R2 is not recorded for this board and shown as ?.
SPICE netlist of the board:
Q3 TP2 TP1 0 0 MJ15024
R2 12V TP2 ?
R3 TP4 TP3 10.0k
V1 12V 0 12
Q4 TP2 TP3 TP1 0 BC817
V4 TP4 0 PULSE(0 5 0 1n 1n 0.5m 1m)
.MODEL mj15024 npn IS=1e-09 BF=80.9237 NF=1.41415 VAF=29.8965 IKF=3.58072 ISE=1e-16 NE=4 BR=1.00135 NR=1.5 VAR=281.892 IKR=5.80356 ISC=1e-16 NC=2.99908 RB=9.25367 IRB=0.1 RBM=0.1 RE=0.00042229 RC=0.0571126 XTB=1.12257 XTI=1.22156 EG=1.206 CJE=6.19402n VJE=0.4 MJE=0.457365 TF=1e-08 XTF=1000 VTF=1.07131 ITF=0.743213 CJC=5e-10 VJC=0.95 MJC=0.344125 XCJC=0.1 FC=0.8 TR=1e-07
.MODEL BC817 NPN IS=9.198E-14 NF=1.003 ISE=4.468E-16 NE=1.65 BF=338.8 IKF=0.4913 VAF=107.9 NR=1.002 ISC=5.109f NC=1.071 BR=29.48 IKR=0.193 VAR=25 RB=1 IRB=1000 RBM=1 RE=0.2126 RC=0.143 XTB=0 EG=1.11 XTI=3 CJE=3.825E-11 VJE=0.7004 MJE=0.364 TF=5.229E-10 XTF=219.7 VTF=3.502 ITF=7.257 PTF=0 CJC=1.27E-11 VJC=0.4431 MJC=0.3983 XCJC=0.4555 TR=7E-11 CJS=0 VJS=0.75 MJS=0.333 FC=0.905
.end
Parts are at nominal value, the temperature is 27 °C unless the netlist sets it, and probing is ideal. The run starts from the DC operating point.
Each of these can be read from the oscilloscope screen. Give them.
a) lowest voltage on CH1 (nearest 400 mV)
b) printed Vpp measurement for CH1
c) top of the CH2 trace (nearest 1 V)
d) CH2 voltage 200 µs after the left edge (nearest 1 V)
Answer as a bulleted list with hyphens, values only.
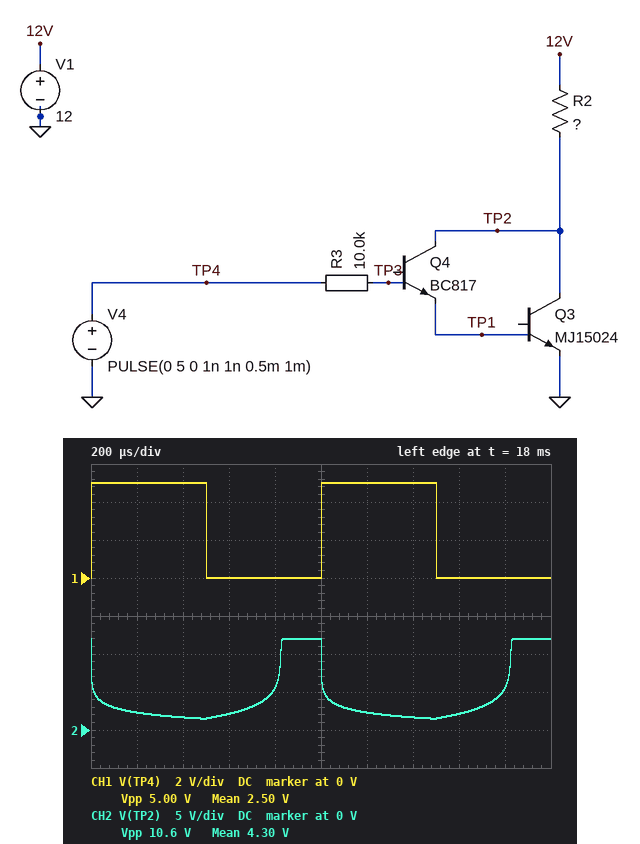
- 0 V
- 5.00 V
- 12 V
- 2 V
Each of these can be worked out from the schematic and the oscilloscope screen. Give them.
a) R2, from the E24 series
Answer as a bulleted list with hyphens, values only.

- 3.6 Ω
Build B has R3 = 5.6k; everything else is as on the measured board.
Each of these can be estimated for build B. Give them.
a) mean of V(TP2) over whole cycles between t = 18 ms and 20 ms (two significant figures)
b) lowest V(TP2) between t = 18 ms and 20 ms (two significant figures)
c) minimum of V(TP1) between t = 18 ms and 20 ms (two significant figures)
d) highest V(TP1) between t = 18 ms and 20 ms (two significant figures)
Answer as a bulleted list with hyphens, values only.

- 3.5 V
- 1.3 V
- 490 mV
- 1.7 V
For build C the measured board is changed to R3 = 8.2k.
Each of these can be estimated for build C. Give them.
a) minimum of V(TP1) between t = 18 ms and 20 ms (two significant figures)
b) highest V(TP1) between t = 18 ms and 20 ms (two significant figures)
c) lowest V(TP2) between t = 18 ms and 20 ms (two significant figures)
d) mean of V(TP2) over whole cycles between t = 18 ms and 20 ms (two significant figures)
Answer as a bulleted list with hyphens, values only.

- 490 mV
- 1.5 V
- 1.3 V
- 3.8 V
